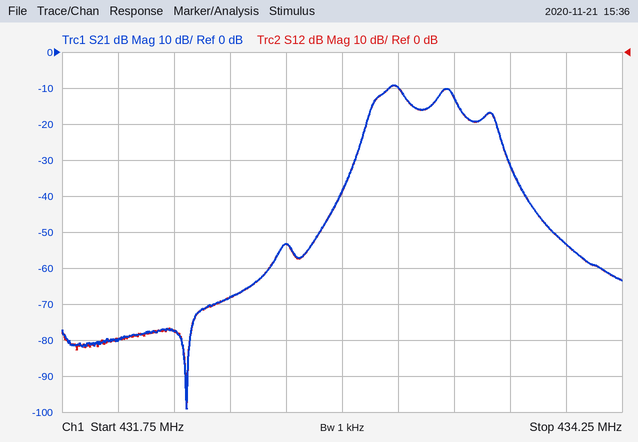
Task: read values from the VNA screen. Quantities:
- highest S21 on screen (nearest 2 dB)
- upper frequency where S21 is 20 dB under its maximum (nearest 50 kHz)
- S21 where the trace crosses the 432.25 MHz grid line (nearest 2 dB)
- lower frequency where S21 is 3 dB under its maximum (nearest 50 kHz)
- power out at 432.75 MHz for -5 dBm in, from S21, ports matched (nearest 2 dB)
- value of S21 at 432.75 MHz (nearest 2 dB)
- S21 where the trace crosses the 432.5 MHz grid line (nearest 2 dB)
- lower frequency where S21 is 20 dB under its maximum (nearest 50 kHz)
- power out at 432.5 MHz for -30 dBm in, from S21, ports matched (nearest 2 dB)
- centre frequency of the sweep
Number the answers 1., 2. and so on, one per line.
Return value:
1. -10 dB
2. 433.75 MHz
3. -78 dB
4. 433.15 MHz
5. -58 dBm
6. -54 dB
7. -68 dB
8. 433.05 MHz
9. -98 dBm
10. 433 MHz
